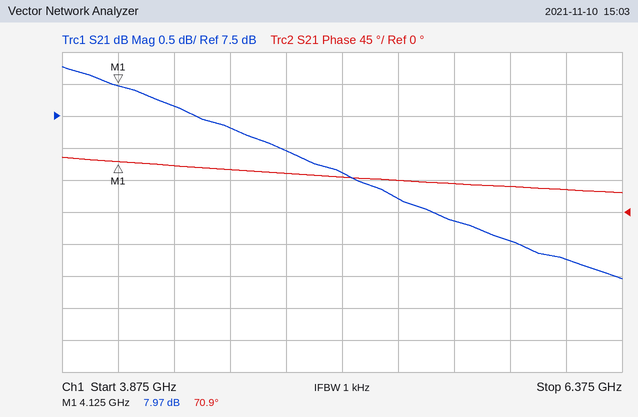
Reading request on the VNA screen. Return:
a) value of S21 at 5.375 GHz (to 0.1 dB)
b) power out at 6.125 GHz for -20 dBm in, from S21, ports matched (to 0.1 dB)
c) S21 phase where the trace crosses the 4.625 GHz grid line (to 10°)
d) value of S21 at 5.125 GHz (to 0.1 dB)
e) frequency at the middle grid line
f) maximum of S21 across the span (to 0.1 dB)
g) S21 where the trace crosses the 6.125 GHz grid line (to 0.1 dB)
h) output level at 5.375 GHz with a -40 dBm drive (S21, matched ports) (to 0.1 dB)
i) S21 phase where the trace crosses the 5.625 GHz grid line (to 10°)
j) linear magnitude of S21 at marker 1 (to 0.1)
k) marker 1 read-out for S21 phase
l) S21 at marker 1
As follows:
6.2 dB
-14.7 dBm
60°
6.6 dB
5.125 GHz
8.3 dB
5.3 dB
-33.8 dBm
40°
2.5
70.9°
7.97 dB
